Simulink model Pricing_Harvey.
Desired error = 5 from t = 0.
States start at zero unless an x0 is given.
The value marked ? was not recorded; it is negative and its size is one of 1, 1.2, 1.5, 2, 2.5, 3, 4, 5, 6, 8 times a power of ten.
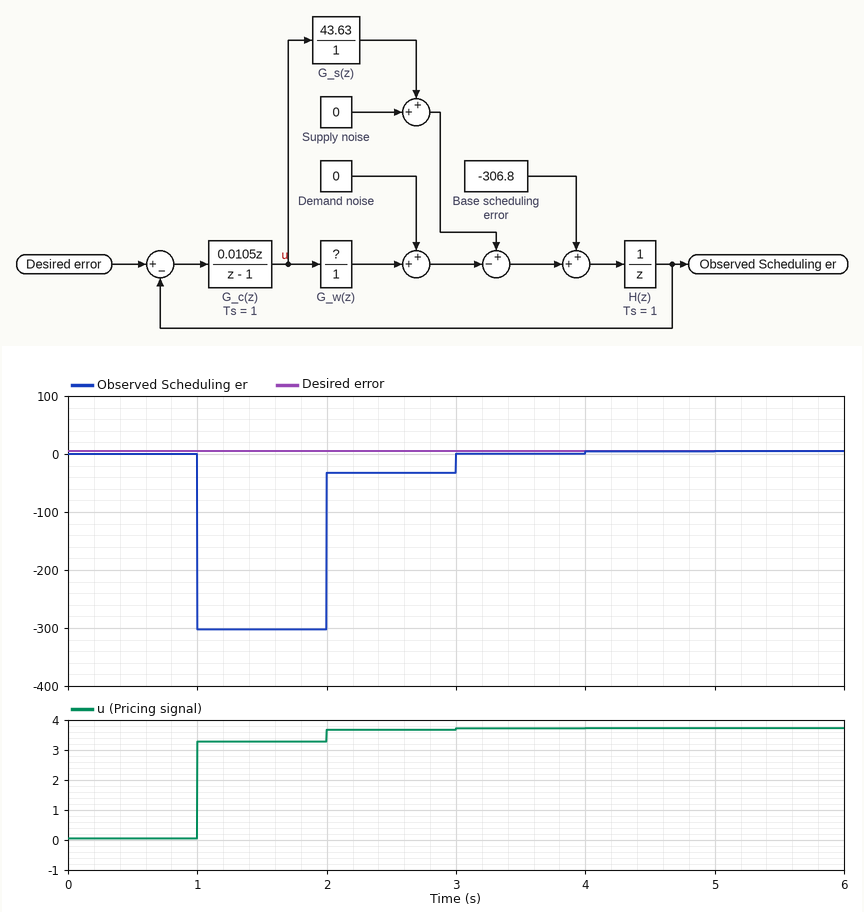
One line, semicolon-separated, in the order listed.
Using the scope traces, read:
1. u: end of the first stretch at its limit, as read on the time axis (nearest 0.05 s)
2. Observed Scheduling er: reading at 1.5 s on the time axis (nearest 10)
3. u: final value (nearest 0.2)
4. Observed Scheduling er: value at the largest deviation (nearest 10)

1.00 s; -300; 3.8; -300
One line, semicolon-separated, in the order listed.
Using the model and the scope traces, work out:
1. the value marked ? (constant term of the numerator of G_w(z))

-40
